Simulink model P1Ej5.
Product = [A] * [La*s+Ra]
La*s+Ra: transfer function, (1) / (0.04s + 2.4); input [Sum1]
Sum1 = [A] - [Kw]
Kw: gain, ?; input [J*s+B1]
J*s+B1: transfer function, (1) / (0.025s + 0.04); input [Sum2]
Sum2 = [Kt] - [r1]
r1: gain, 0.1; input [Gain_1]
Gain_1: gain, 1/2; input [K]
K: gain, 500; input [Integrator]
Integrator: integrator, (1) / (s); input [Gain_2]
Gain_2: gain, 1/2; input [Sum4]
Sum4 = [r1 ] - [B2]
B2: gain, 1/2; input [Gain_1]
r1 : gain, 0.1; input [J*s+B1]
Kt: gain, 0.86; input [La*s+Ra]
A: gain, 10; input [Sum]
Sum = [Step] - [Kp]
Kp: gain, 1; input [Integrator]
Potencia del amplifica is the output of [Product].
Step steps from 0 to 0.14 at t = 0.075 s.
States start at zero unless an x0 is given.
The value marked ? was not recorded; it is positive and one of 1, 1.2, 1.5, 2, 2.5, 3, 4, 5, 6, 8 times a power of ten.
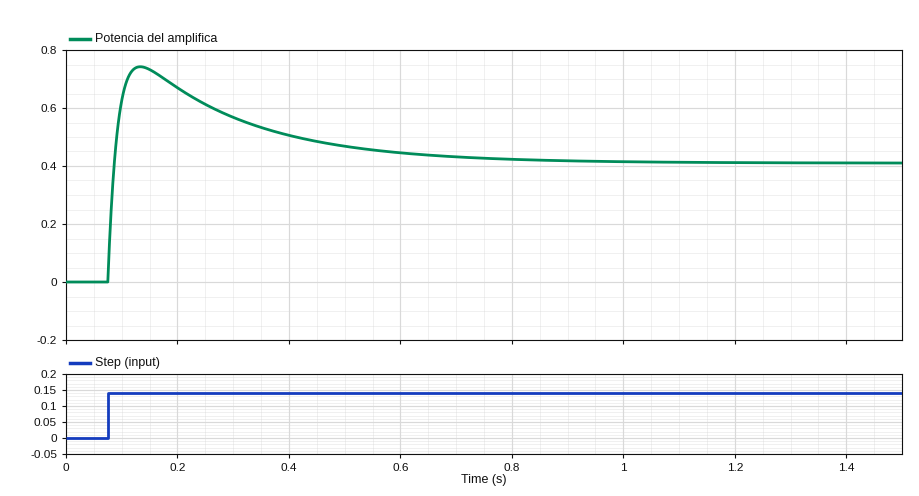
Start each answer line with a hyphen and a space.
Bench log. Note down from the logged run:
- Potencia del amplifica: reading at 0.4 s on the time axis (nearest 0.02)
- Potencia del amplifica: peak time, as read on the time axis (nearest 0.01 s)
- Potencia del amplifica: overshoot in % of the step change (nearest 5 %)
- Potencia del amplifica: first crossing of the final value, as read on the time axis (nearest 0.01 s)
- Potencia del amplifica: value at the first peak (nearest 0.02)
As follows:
- 0.50
- 0.13 s
- 80 %
- 0.09 s
- 0.74
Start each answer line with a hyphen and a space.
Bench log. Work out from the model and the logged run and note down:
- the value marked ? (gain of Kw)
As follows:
- 0.15
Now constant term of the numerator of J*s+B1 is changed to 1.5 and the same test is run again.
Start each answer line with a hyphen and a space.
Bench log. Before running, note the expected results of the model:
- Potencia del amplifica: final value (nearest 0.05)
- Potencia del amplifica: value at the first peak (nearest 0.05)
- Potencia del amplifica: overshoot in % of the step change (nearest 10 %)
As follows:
- 0.35
- 0.70
- 100 %
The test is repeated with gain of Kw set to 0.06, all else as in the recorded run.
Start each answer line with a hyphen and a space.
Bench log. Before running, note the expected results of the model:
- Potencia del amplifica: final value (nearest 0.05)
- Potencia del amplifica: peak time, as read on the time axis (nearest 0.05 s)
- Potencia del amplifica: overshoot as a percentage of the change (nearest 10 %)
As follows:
- 0.55
- 0.15 s
- 40 %
